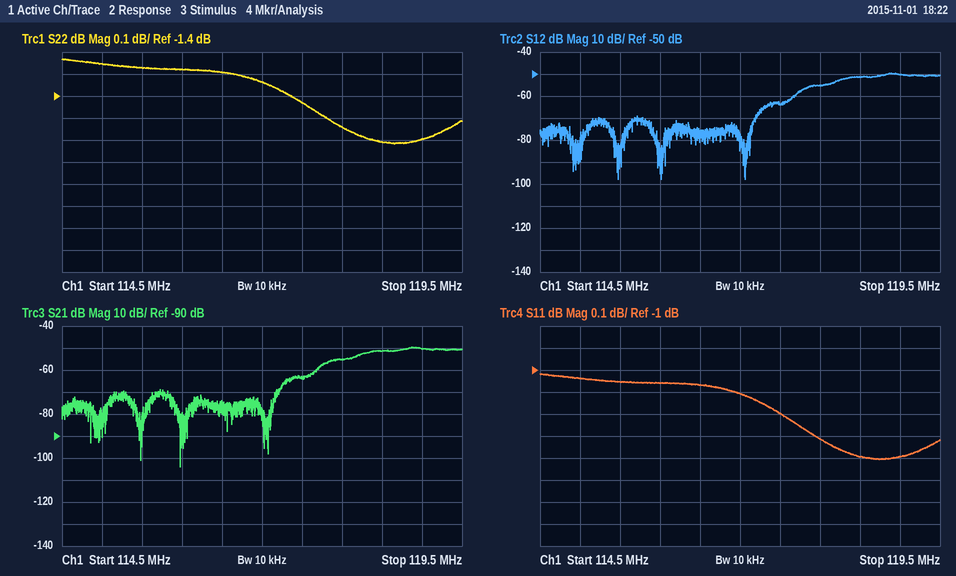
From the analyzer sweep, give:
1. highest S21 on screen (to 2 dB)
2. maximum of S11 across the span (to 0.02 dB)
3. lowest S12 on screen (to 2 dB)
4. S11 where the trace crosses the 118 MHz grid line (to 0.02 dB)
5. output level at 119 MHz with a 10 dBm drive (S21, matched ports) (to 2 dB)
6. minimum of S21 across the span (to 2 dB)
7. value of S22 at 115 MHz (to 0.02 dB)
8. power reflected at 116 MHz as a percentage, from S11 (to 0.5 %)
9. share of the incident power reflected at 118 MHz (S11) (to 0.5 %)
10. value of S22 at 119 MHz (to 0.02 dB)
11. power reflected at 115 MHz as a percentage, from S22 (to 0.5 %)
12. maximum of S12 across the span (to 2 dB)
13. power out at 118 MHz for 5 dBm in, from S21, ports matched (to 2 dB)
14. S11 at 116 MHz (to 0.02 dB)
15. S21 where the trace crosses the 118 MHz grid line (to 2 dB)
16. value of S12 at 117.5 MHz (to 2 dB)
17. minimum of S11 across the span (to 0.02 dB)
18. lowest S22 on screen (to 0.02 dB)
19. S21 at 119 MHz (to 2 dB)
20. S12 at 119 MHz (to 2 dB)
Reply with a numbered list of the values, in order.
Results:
1. -50 dB
2. -1.02 dB
3. -98 dB
4. -1.32 dB
5. -40 dBm
6. -104 dB
7. -1.26 dB
8. 78.5 %
9. 74.0 %
10. -1.60 dB
11. 75.0 %
12. -50 dB
13. -50 dBm
14. -1.06 dB
15. -56 dB
16. -64 dB
17. -1.40 dB
18. -1.62 dB
19. -50 dB
20. -50 dB
